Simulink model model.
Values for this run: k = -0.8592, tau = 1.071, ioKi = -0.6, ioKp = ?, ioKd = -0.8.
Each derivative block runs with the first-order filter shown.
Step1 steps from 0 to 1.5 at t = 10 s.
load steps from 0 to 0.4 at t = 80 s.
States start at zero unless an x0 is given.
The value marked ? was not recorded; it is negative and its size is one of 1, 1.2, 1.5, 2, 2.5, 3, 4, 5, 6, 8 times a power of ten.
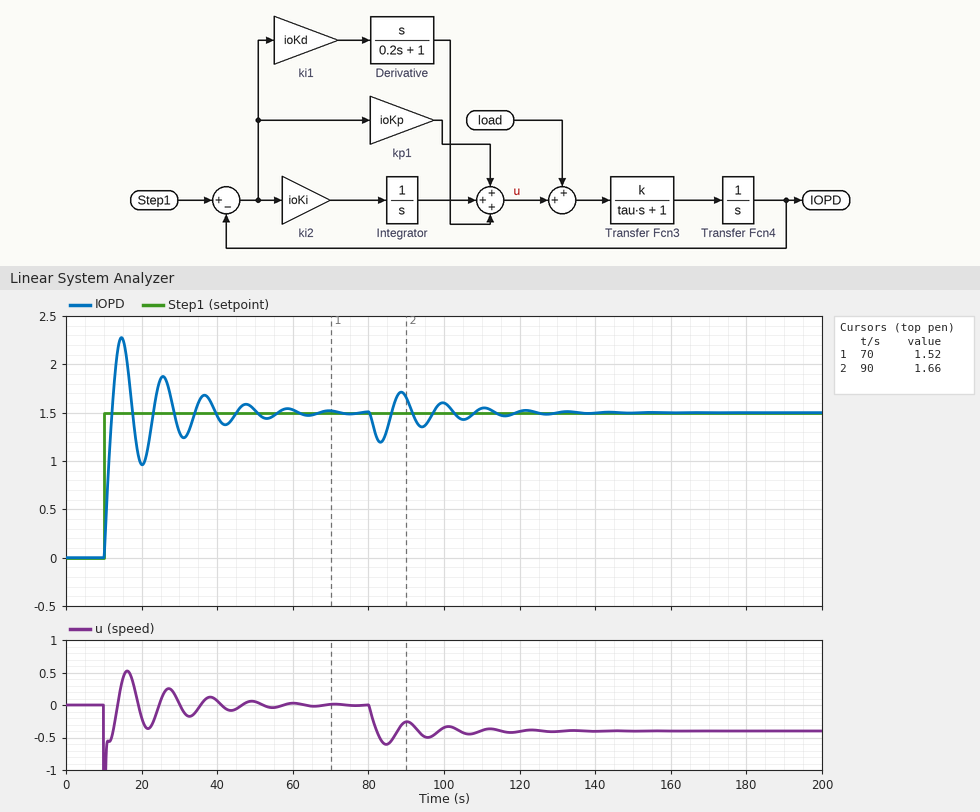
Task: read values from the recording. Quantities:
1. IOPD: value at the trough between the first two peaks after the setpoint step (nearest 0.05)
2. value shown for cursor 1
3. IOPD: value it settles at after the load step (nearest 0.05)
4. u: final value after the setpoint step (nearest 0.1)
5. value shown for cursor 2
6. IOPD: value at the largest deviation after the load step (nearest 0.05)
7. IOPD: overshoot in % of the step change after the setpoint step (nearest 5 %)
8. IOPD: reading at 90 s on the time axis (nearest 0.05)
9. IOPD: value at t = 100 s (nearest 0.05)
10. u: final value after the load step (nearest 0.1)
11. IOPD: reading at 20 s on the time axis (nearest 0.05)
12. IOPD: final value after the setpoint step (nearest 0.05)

0.95
1.52
1.50
0.0
1.66
1.20
50 %
1.65
1.60
-0.4
0.95
1.50
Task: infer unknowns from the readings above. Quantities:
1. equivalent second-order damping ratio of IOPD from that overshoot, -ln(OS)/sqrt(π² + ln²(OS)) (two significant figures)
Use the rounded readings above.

0.22
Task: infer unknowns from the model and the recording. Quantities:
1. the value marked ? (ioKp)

-0.6
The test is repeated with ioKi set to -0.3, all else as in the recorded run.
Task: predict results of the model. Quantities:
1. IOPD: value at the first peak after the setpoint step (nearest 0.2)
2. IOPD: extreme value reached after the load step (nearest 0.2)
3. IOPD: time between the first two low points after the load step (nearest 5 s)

2.0
1.2
15 s
